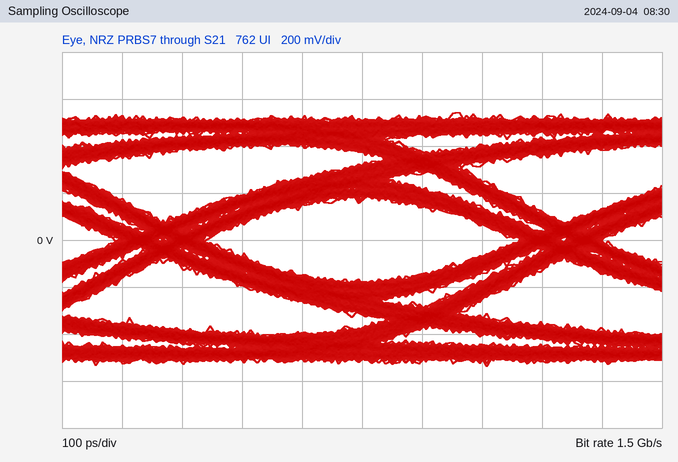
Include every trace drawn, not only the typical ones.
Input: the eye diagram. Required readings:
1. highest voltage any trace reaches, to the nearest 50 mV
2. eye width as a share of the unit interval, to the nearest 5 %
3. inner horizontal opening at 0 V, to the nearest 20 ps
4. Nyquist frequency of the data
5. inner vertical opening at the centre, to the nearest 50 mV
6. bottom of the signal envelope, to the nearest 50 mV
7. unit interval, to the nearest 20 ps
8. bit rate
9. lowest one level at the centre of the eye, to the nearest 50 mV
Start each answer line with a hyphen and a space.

- 550 mV
- 80 %
- 520 ps
- 750 MHz
- 350 mV
- -550 mV
- 660 ps
- 1.5 Gb/s
- 150 mV
